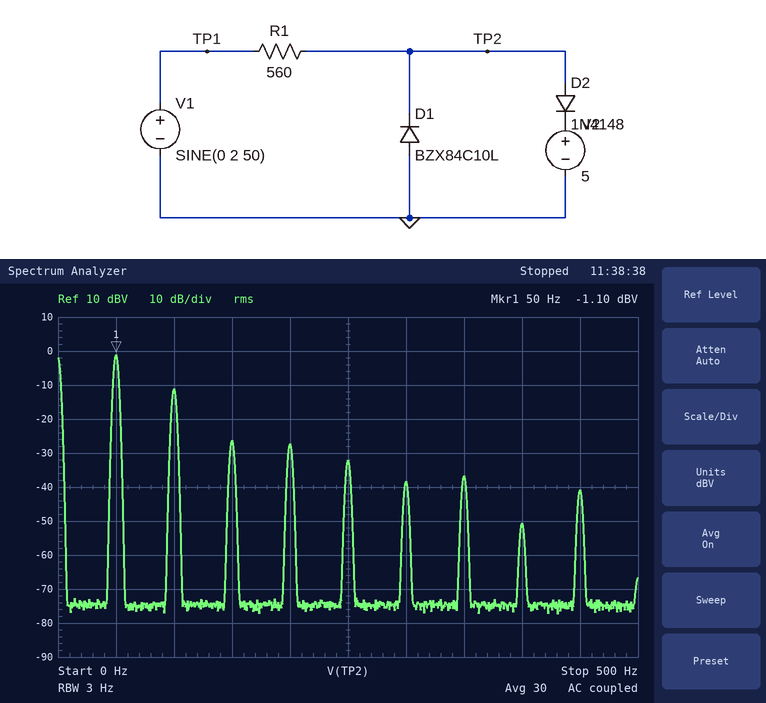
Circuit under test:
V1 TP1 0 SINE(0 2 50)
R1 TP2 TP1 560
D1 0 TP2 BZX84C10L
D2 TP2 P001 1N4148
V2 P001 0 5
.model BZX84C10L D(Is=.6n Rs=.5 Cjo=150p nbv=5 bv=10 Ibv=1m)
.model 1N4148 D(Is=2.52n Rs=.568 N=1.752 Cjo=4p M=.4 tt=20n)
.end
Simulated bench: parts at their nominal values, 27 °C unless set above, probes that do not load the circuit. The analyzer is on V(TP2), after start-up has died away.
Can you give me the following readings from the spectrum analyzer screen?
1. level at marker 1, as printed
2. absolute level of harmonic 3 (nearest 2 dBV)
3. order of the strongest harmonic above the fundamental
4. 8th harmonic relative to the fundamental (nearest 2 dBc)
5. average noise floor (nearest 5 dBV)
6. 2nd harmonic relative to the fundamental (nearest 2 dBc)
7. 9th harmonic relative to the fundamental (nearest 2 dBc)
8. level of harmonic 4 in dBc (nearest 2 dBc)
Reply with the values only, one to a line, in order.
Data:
-1.10 dBV
-26 dBV
2
-50 dBc
-75 dBV
-10 dBc
-40 dBc
-26 dBc
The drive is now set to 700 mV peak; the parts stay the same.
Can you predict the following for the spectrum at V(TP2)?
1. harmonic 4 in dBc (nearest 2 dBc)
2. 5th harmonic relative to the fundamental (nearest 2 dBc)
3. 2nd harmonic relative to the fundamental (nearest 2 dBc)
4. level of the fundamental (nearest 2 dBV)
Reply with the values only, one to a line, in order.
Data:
-44 dBc
-36 dBc
-16 dBc
-8 dBV
